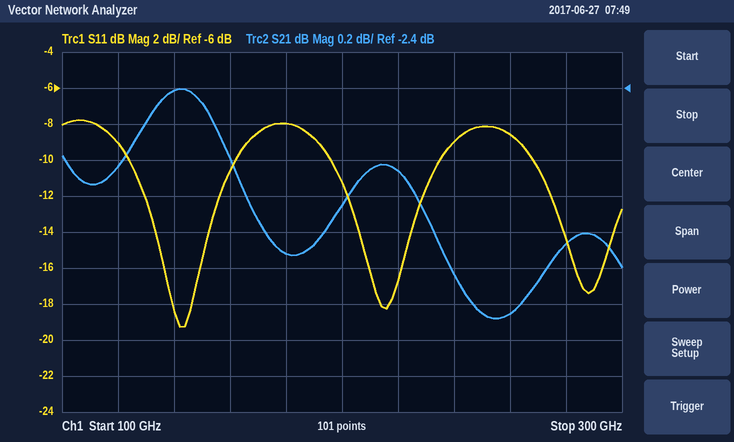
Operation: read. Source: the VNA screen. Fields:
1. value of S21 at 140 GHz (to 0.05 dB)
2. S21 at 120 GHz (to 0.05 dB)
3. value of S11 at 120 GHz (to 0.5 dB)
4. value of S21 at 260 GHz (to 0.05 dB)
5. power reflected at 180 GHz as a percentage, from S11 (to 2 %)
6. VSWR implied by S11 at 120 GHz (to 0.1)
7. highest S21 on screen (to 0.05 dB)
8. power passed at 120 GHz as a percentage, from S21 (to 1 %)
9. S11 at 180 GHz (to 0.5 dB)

-2.40 dB
-2.85 dB
-9.0 dB
-3.65 dB
16 %
2.1
-2.40 dB
52 %
-8.0 dB
